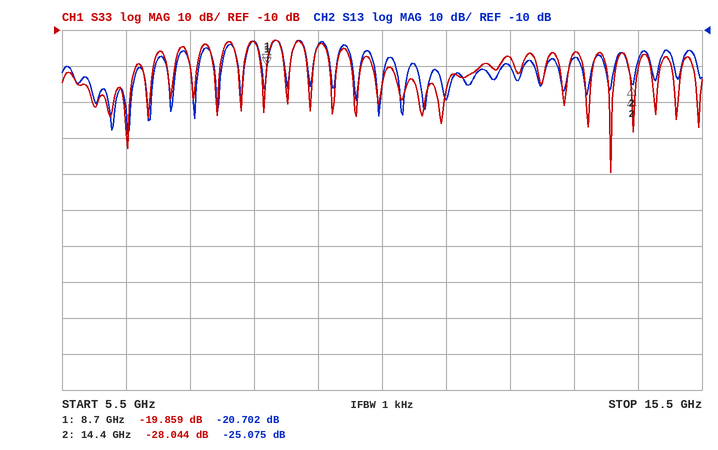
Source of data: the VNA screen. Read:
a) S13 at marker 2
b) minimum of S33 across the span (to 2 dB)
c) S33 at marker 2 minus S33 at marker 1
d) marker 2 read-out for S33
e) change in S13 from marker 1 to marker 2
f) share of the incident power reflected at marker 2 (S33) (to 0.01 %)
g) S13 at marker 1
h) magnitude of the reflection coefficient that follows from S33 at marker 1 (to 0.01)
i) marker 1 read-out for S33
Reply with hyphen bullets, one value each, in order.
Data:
- -25.075 dB
- -50 dB
- -8.185 dB
- -28.044 dB
- -4.373 dB
- 0.16 %
- -20.702 dB
- 0.10
- -19.859 dB
